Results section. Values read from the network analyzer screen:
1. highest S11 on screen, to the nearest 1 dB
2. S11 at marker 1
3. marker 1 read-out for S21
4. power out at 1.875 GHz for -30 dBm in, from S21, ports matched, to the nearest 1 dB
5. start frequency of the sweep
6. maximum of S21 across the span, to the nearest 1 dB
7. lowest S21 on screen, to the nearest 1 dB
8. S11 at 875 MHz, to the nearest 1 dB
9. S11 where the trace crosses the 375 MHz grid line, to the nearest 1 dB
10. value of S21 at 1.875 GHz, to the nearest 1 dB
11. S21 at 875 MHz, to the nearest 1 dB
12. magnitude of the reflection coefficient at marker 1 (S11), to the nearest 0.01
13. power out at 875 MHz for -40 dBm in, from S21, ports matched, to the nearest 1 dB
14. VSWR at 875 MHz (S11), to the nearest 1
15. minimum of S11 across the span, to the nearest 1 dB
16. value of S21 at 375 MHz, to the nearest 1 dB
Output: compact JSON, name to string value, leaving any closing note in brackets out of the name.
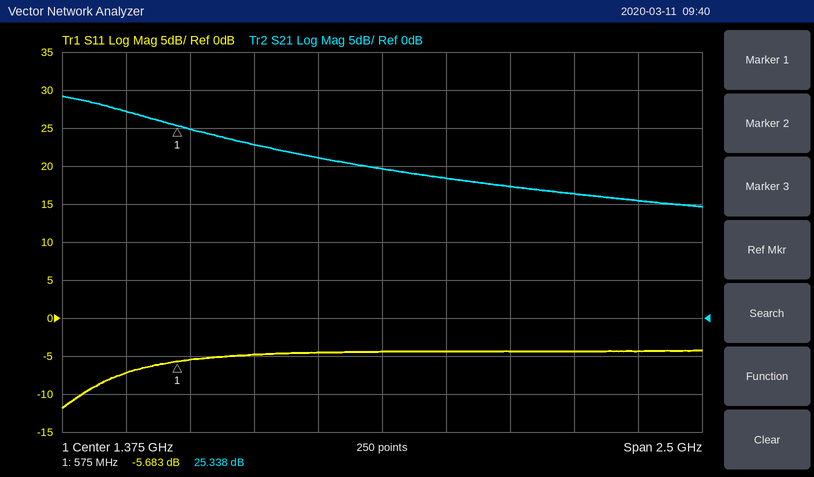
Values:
{"highest S11 on screen, to the nearest 1 dB": "-4 dB", "S11 at marker 1": "-5.683 dB", "marker 1 read-out for S21": "25.338 dB", "power out at 1.875 GHz for -30 dBm in, from S21, ports matched, to the nearest 1 dB": "-13 dBm", "start frequency of the sweep": "125 MHz", "maximum of S21 across the span, to the nearest 1 dB": "29 dB", "lowest S21 on screen, to the nearest 1 dB": "15 dB", "S11 at 875 MHz, to the nearest 1 dB": "-5 dB", "S11 where the trace crosses the 375 MHz grid line, to the nearest 1 dB": "-7 dB", "value of S21 at 1.875 GHz, to the nearest 1 dB": "17 dB", "S21 at 875 MHz, to the nearest 1 dB": "23 dB", "magnitude of the reflection coefficient at marker 1 (S11), to the nearest 0.01": "0.52", "power out at 875 MHz for -40 dBm in, from S21, ports matched, to the nearest 1 dB": "-17 dBm", "VSWR at 875 MHz (S11), to the nearest 1": "4", "minimum of S11 across the span, to the nearest 1 dB": "-12 dB", "value of S21 at 375 MHz, to the nearest 1 dB": "27 dB"}
